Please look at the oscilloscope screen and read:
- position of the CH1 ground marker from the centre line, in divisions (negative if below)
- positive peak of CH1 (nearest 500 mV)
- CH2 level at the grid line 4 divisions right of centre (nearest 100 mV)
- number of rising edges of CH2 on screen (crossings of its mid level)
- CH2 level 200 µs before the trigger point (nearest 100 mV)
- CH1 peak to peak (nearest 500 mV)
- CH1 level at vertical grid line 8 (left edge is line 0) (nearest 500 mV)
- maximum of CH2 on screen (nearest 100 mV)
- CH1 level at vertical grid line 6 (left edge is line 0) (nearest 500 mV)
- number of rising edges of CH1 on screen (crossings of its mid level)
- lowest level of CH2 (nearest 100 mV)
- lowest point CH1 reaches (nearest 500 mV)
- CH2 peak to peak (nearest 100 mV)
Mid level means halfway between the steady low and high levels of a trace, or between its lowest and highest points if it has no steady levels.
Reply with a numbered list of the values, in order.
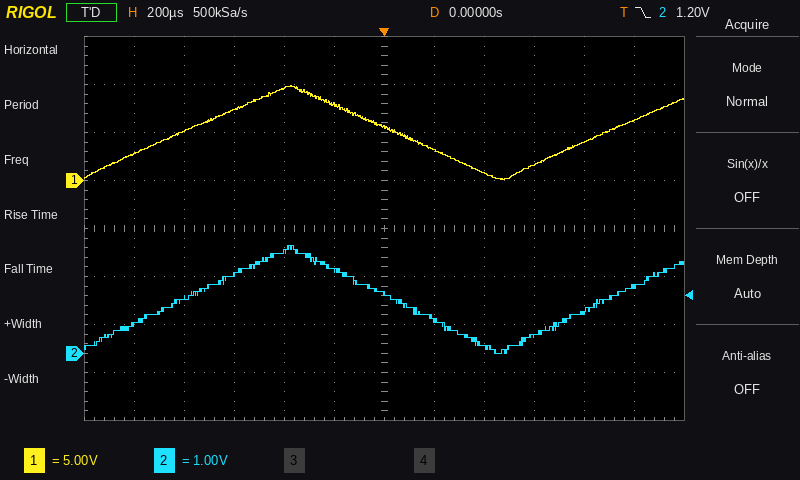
1. +1.0 div
2. 10.0 V
3. 900 mV
4. 2
5. 1.7 V
6. 10.0 V
7. 1.0 V
8. 2.2 V
9. 5.5 V
10. 2
11. 0.0 V
12. 0.0 V
13. 2.2 V
